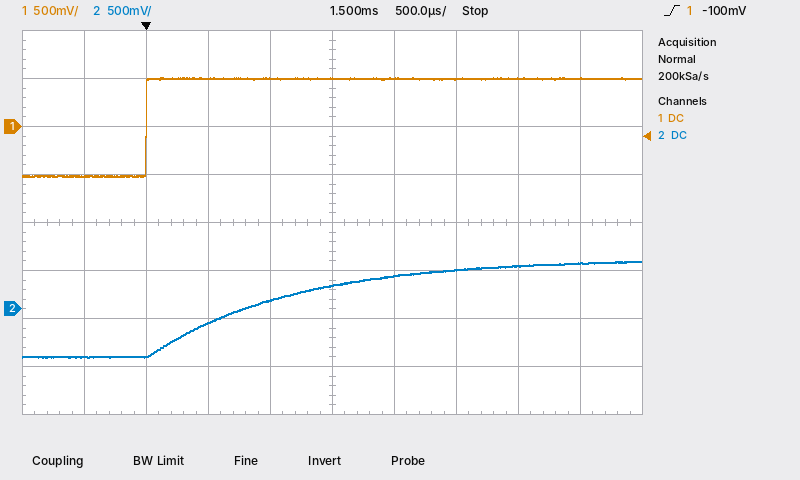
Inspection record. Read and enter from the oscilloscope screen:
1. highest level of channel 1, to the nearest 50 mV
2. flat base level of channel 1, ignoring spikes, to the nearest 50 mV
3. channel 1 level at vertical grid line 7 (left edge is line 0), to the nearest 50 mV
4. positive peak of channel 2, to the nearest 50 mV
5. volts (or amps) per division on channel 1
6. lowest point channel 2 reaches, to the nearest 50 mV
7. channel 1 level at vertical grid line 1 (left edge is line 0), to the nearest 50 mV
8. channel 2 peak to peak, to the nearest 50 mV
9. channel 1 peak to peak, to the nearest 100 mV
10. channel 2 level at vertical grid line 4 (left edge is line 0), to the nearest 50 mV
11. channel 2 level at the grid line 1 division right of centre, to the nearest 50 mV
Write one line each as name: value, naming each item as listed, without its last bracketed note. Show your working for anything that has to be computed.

highest level of channel 1, to the nearest 50 mV: 500 mV
flat base level of channel 1, ignoring spikes, to the nearest 50 mV: -500 mV
channel 1 level at vertical grid line 7 (left edge is line 0), to the nearest 50 mV: 500 mV
positive peak of channel 2, to the nearest 50 mV: 500 mV
volts (or amps) per division on channel 1: 500 mV
lowest point channel 2 reaches, to the nearest 50 mV: -500 mV
channel 1 level at vertical grid line 1 (left edge is line 0), to the nearest 50 mV: -500 mV
channel 2 peak to peak, to the nearest 50 mV: 500 mV − (-500 mV) = 1.00 V
channel 1 peak to peak, to the nearest 100 mV: 1.00 V
channel 2 level at vertical grid line 4 (left edge is line 0), to the nearest 50 mV: 100 mV
channel 2 level at the grid line 1 division right of centre, to the nearest 50 mV: 350 mV
